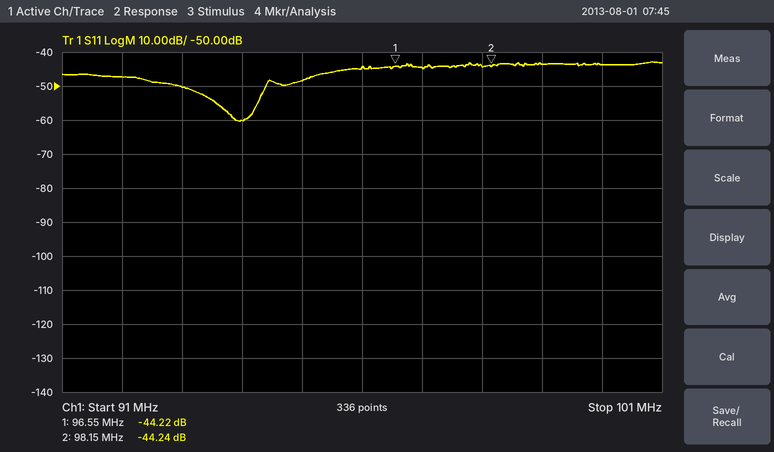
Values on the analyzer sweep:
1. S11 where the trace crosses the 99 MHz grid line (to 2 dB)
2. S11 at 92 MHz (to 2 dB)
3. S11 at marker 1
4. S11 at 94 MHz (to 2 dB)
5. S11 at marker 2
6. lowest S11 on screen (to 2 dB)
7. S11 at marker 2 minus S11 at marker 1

-44 dB
-48 dB
-44.22 dB
-60 dB
-44.24 dB
-60 dB
-0.02 dB
